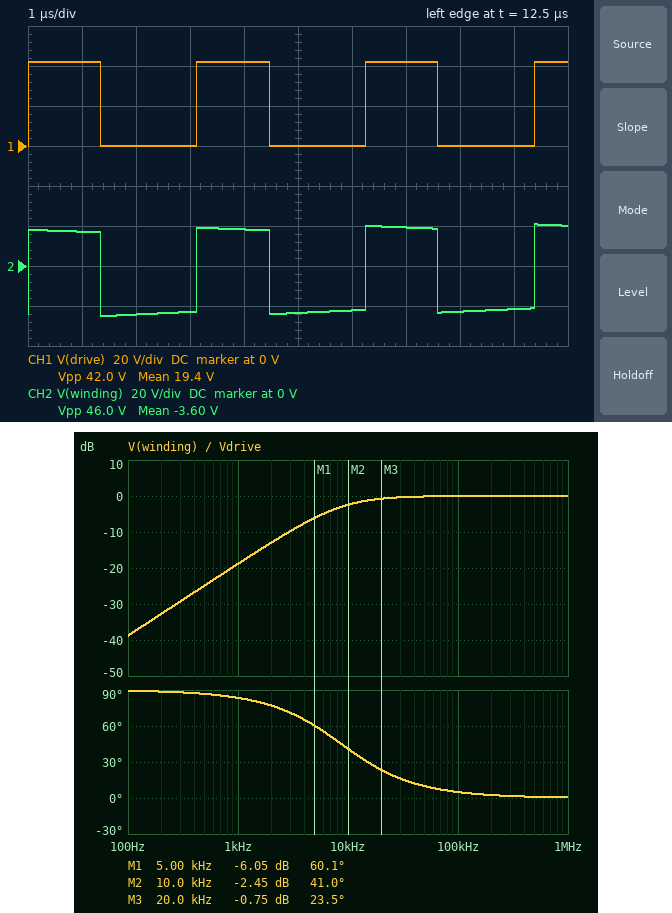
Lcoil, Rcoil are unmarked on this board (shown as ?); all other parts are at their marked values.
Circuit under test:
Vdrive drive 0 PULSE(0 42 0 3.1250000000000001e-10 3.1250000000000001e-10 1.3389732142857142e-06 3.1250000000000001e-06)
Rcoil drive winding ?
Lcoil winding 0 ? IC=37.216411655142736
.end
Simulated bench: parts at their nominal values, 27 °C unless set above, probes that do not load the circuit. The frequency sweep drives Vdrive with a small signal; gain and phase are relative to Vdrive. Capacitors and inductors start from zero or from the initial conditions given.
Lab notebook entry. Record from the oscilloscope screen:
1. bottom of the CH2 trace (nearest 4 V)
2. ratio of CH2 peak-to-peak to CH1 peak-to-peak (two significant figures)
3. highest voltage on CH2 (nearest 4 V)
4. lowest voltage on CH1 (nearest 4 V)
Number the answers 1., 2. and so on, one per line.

1. -24 V
2. 1.1
3. 20 V
4. 0 V
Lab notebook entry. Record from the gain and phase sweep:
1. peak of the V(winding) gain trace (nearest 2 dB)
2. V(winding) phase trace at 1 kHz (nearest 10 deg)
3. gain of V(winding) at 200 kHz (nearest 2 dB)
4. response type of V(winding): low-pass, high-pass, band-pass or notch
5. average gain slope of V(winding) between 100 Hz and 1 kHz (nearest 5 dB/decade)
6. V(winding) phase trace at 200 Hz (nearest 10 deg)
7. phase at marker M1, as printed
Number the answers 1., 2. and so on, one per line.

1. 0 dB
2. 80 deg
3. 0 dB
4. high-pass
5. 20 dB/decade
6. 90 deg
7. 60.1 deg
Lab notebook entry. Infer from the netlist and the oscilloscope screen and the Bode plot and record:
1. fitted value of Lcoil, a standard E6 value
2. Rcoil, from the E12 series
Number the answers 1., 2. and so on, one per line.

1. 15 µH
2. 0.82 Ω
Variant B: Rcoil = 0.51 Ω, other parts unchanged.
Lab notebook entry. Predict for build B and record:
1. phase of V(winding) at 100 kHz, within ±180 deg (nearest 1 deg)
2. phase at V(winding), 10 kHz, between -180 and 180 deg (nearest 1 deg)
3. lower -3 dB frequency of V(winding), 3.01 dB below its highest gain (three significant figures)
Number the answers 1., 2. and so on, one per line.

1. 3 deg
2. 28 deg
3. 5.41 kHz
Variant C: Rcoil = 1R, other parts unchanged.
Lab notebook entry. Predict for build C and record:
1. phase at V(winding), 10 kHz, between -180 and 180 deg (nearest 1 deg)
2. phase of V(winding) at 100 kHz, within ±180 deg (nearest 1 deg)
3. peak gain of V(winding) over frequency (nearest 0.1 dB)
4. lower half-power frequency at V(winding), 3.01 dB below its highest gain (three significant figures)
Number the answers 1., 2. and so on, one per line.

1. 47 deg
2. 6 deg
3. 0 dB
4. 10.6 kHz
